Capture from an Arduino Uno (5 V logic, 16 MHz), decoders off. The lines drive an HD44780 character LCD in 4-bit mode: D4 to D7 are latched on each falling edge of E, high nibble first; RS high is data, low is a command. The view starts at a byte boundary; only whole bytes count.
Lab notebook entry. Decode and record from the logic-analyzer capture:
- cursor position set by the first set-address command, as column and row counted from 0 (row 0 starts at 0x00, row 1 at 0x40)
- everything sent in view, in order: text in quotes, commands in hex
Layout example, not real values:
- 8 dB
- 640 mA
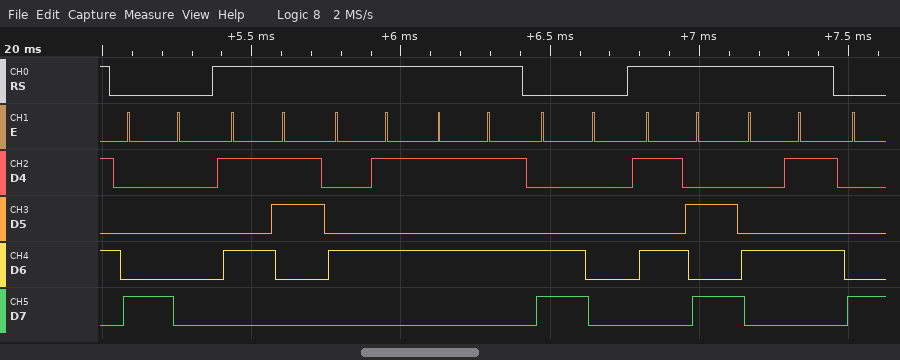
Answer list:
- column 0, row 0
- 0x80 "SEU" 0xC0 "ZE"
